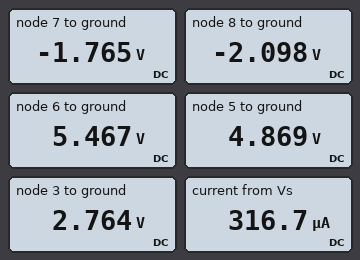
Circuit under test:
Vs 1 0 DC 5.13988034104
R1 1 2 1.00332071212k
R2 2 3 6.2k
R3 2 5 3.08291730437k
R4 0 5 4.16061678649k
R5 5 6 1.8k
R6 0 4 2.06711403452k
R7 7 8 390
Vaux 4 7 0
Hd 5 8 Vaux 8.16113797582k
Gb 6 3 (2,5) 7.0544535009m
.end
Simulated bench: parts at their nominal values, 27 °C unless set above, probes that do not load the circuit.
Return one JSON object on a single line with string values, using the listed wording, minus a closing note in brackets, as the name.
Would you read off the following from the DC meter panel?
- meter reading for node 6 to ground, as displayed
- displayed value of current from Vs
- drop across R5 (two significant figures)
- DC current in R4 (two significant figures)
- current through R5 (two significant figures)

{"meter reading for node 6 to ground, as displayed": "5.467 V", "displayed value of current from Vs": "316.7 µA", "drop across R5": "600 mV", "DC current in R4": "1.2 mA", "current through R5": "330 µA"}
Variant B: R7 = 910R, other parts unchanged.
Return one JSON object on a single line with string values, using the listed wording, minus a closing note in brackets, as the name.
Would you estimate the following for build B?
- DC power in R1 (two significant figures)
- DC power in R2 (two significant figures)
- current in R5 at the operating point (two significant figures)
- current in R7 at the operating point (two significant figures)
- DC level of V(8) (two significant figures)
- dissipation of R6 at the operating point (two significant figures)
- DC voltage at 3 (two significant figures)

{"DC power in R1": "55 µW", "DC power in R2": "370 µW", "current in R5 at the operating point": "250 µA", "current in R7 at the operating point": "950 µA", "DC level of V(8)": "-2.8 V", "dissipation of R6 at the operating point": "1.9 mW", "DC voltage at 3": "3.4 V"}
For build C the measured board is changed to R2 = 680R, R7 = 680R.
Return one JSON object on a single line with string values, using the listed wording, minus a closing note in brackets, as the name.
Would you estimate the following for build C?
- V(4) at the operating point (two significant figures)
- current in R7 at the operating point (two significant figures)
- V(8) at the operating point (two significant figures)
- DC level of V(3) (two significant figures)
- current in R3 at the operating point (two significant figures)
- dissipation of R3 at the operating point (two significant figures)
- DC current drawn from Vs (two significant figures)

{"V(4) at the operating point": "-1.9 V", "current in R7 at the operating point": "910 µA", "V(8) at the operating point": "-2.5 V", "DC level of V(3)": "4.7 V", "current in R3 at the operating point": "13 µA", "dissipation of R3 at the operating point": "530 nW", "DC current drawn from Vs": "270 µA"}
